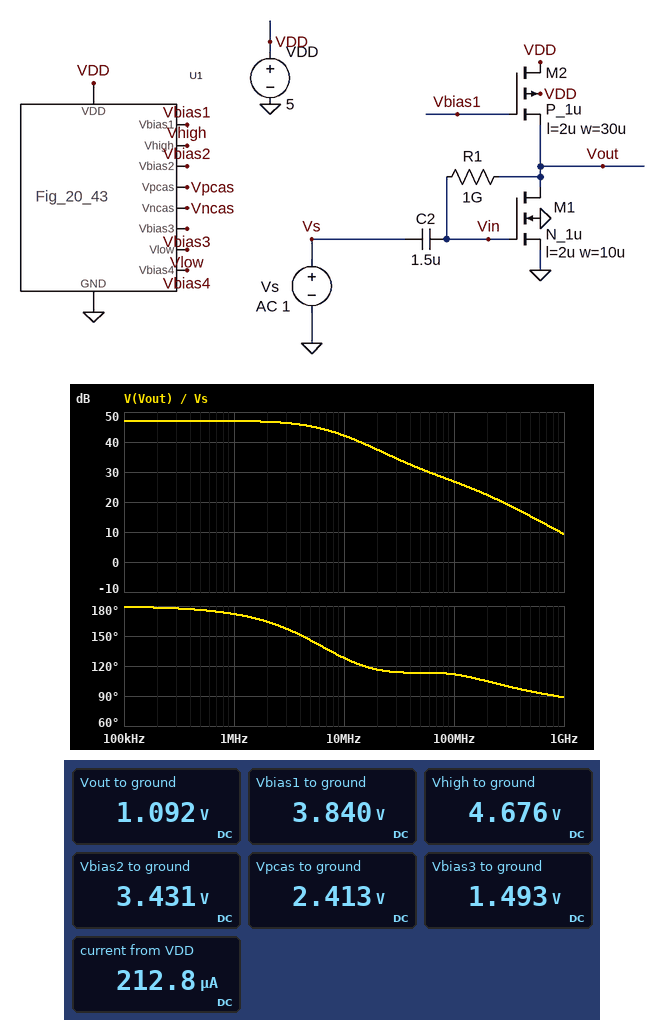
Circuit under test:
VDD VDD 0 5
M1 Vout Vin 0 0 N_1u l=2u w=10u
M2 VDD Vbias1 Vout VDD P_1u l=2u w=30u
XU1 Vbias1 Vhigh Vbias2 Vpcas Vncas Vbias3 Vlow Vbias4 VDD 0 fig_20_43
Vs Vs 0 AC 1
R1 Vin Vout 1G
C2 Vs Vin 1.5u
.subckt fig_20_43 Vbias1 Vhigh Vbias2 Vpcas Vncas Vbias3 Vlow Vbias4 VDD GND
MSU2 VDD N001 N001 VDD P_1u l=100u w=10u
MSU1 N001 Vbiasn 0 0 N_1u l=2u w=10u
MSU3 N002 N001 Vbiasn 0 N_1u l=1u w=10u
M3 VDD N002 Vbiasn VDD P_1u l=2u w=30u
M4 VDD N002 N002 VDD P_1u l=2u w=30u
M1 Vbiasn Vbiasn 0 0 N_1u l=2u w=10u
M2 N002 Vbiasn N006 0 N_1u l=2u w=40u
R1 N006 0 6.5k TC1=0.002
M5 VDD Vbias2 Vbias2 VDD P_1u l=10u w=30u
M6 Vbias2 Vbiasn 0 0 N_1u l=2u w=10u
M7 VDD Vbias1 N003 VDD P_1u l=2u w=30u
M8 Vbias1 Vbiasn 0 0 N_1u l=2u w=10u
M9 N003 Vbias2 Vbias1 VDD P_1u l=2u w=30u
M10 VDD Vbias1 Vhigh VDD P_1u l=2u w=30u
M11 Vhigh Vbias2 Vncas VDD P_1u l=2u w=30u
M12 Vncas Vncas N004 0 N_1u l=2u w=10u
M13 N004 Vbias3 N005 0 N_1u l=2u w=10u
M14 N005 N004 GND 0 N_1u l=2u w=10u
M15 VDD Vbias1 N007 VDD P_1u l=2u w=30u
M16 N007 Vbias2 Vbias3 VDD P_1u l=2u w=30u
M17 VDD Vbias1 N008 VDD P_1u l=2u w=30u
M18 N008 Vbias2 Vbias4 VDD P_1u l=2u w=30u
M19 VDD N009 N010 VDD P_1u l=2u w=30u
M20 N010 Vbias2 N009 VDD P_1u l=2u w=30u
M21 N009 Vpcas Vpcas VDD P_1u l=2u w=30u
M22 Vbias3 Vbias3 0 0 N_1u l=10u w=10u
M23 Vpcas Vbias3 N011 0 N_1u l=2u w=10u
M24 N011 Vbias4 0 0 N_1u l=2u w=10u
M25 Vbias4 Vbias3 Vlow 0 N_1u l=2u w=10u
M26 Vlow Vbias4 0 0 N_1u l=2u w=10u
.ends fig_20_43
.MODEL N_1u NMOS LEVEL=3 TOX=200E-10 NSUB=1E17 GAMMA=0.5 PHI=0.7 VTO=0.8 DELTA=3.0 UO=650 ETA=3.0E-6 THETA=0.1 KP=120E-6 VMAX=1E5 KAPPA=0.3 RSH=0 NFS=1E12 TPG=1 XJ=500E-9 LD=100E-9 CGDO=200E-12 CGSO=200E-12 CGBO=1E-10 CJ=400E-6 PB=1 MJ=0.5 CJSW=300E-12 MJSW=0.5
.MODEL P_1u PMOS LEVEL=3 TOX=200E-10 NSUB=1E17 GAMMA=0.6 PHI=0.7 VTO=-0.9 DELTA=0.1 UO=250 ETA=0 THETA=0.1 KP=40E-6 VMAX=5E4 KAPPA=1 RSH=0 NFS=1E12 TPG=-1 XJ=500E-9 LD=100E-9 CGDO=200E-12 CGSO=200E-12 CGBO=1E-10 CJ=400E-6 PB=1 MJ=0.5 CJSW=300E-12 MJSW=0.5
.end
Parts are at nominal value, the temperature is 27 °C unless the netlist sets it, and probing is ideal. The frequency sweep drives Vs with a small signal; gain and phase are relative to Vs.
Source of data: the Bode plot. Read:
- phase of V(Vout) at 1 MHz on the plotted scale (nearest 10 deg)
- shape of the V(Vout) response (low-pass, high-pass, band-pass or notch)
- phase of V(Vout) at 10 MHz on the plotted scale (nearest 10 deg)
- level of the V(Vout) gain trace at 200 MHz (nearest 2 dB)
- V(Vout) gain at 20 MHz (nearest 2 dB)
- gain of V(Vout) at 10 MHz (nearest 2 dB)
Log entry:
170 deg
low-pass
130 deg
22 dB
38 dB
42 dB
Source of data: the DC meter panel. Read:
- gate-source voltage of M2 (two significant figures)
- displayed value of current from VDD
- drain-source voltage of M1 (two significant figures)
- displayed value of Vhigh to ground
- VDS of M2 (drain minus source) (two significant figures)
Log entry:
2.7 V
212.8 µA
1.1 V
4.676 V
3.9 V
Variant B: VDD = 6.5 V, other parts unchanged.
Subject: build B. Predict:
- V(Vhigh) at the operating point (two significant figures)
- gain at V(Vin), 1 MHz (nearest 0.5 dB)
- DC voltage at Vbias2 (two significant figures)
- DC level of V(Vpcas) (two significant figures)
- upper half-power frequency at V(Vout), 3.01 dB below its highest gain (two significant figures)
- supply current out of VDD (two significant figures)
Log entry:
6.2 V
0 dB
4.9 V
3.9 V
7.2 MHz
230 µA
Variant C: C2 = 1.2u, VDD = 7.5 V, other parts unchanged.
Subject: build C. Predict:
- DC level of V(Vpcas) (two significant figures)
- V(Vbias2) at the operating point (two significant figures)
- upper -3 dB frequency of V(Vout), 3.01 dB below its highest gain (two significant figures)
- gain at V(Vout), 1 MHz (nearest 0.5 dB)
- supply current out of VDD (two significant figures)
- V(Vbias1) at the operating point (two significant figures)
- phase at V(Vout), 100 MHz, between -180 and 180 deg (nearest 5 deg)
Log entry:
4.9 V
5.9 V
7.9 MHz
46.5 dB
250 µA
6.3 V
115 deg
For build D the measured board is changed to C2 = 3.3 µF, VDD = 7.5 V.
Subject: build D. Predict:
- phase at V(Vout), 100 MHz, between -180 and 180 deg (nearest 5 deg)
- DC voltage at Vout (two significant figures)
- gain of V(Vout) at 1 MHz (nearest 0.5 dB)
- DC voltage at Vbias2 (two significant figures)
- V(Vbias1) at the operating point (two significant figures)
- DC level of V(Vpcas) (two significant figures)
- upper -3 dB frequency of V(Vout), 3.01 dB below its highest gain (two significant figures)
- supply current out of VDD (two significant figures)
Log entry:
115 deg
1.1 V
46.5 dB
5.9 V
6.3 V
4.9 V
7.9 MHz
250 µA
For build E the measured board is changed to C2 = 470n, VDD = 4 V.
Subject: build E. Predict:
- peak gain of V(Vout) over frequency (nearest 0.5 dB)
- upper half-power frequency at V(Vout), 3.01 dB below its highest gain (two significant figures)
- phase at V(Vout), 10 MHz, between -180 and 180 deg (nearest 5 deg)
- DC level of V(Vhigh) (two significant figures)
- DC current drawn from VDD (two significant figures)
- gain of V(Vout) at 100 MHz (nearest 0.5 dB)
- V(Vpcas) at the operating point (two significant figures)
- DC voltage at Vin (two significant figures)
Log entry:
47.5 dB
6.5 MHz
125 deg
3.7 V
200 µA
26.5 dB
1.4 V
1.1 V
